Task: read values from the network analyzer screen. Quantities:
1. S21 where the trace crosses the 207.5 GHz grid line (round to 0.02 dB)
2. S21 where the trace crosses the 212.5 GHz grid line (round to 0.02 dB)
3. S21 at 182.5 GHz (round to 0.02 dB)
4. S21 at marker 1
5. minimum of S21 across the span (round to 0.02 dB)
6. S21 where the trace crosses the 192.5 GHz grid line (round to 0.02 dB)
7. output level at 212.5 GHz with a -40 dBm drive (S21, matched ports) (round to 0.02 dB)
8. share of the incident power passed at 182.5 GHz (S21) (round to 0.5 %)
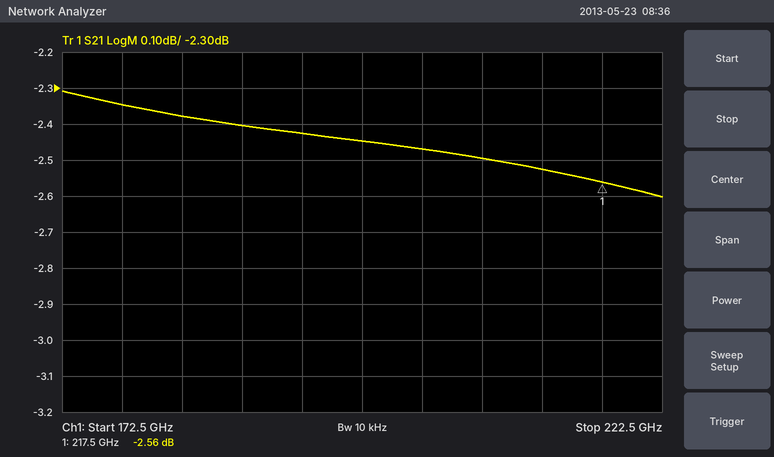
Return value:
-2.50 dB
-2.52 dB
-2.38 dB
-2.56 dB
-2.60 dB
-2.42 dB
-42.52 dBm
58.0 %
